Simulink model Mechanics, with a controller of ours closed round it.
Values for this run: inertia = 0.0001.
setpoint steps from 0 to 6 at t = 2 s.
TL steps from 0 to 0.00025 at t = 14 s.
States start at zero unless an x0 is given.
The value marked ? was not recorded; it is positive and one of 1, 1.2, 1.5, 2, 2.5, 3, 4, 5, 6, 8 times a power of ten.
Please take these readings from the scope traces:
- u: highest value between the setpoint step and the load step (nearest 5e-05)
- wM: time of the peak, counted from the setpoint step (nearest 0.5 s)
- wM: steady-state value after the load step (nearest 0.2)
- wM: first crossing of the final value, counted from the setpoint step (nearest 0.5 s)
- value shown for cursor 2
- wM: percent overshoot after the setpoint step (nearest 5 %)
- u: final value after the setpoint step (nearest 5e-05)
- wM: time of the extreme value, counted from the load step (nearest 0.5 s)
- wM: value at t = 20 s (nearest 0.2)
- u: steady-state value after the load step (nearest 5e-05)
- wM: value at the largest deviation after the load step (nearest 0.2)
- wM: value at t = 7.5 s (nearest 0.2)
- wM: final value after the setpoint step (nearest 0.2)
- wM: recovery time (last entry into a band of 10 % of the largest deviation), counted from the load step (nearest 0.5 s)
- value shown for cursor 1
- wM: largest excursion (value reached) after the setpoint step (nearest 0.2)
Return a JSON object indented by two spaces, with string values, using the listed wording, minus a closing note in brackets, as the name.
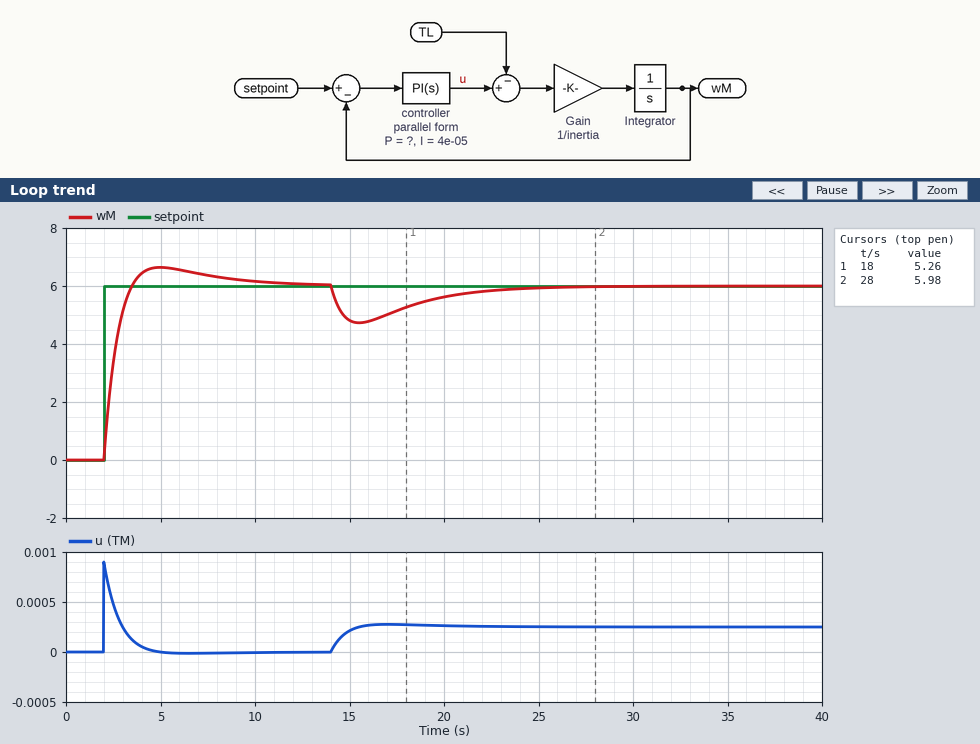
{
  "u: highest value between the setpoint step and the load step": "0.00090",
  "wM: time of the peak, counted from the setpoint step": "3.0 s",
  "wM: steady-state value after the load step": "6.0",
  "wM: first crossing of the final value, counted from the setpoint step": "1.5 s",
  "value shown for cursor 2": "5.98",
  "wM: percent overshoot after the setpoint step": "10 %",
  "u: final value after the setpoint step": "0.00000",
  "wM: time of the extreme value, counted from the load step": "1.5 s",
  "wM: value at t = 20 s": "5.6",
  "u: steady-state value after the load step": "0.00025",
  "wM: value at the largest deviation after the load step": "4.8",
  "wM: value at t = 7.5 s": "6.4",
  "wM: final value after the setpoint step": "6.0",
  "wM: recovery time (last entry into a band of 10 % of the largest deviation), counted from the load step": "9.0 s",
  "value shown for cursor 1": "5.26",
  "wM: largest excursion (value reached) after the setpoint step": "6.6"
}
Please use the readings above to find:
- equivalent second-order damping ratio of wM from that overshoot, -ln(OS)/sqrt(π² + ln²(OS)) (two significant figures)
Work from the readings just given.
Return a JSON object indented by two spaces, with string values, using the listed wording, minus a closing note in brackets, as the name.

{
  "equivalent second-order damping ratio of wM from that overshoot, -ln(OS)/sqrt(π² + ln²(OS))": "0.59"
}
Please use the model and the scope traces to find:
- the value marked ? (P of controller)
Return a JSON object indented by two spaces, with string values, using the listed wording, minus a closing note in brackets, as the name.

{
  "the value marked ?": "0.00015"
}
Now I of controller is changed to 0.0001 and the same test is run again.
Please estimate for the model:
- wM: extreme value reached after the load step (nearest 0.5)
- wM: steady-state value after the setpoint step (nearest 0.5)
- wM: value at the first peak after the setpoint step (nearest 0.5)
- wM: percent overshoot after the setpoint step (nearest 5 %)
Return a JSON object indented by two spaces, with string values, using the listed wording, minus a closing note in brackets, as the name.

{
  "wM: extreme value reached after the load step": "5.0",
  "wM: steady-state value after the setpoint step": "6.0",
  "wM: value at the first peak after the setpoint step": "7.0",
  "wM: percent overshoot after the setpoint step": "20 %"
}
